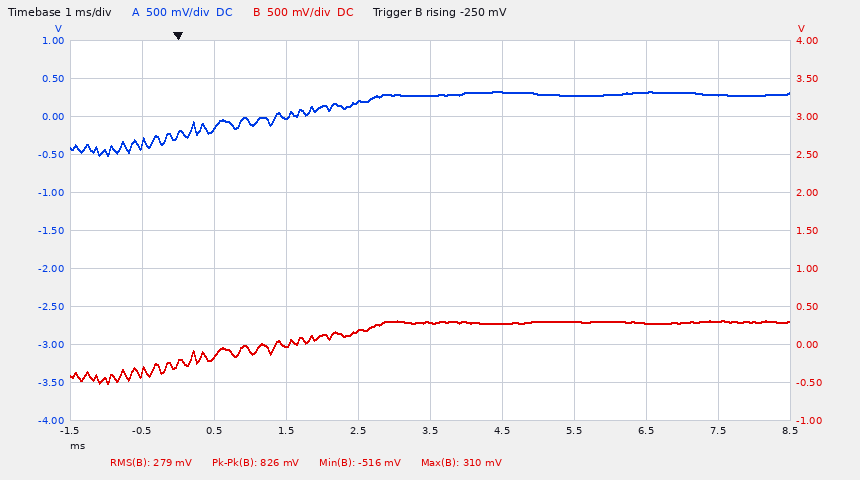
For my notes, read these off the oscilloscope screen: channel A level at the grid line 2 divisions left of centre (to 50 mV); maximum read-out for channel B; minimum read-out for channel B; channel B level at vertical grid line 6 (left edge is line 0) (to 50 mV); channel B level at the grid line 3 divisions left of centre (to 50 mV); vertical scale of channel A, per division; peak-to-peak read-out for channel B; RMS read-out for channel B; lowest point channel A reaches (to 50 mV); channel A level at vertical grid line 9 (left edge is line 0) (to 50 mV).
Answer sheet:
0 mV
310 mV
-516 mV
300 mV
-150 mV
500 mV
826 mV
279 mV
-500 mV
300 mV
